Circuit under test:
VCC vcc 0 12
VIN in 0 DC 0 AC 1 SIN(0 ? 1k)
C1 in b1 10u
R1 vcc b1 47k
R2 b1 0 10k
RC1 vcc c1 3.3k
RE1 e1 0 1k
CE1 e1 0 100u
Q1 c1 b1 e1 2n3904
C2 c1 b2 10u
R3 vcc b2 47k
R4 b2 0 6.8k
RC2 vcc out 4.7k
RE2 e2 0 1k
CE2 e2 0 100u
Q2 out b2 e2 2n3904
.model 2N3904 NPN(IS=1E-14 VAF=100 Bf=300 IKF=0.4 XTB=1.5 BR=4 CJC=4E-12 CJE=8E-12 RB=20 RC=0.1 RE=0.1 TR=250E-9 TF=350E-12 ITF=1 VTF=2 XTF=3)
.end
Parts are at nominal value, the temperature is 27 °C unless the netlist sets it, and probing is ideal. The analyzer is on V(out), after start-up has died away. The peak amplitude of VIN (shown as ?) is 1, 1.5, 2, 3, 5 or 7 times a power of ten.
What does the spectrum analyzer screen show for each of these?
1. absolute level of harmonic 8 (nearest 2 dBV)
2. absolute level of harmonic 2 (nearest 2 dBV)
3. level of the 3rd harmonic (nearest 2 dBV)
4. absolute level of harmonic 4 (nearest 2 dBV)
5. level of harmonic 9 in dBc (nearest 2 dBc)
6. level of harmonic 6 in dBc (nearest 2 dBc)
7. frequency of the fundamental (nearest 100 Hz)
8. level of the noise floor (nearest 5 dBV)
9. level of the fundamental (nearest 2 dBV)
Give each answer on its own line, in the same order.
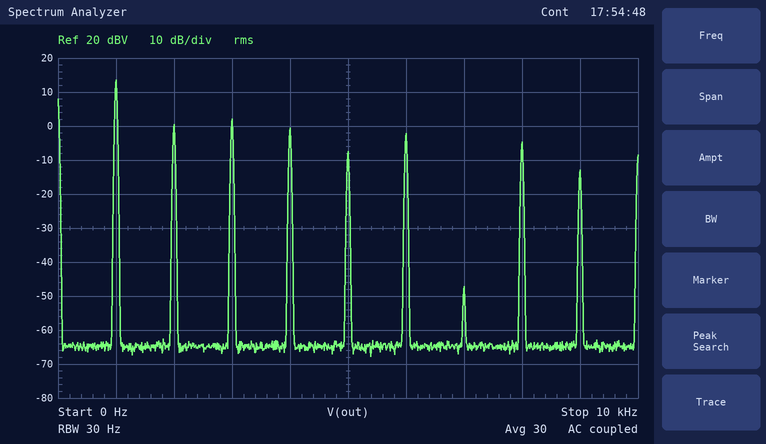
-4 dBV
0 dBV
2 dBV
0 dBV
-26 dBc
-16 dBc
1.0 kHz
-65 dBV
14 dBV
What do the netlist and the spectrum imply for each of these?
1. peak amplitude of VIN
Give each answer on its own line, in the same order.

20 mV
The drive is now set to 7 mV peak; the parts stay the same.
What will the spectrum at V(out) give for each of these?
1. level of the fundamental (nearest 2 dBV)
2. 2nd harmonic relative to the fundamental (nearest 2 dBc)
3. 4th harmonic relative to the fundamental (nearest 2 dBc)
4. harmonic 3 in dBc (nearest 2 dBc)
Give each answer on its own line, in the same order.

14 dBV
-10 dBc
-12 dBc
-14 dBc
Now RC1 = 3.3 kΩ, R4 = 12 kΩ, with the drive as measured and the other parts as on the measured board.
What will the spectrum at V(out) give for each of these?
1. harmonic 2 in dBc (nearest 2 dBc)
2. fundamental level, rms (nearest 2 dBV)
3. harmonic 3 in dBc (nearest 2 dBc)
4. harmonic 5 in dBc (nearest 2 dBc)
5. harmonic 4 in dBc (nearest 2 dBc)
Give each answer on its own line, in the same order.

-20 dBc
14 dBV
-10 dBc
-16 dBc
-20 dBc
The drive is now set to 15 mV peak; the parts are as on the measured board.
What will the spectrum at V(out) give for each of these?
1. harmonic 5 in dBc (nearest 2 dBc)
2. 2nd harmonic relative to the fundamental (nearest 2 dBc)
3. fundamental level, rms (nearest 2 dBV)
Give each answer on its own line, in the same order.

-26 dBc
-12 dBc
14 dBV
